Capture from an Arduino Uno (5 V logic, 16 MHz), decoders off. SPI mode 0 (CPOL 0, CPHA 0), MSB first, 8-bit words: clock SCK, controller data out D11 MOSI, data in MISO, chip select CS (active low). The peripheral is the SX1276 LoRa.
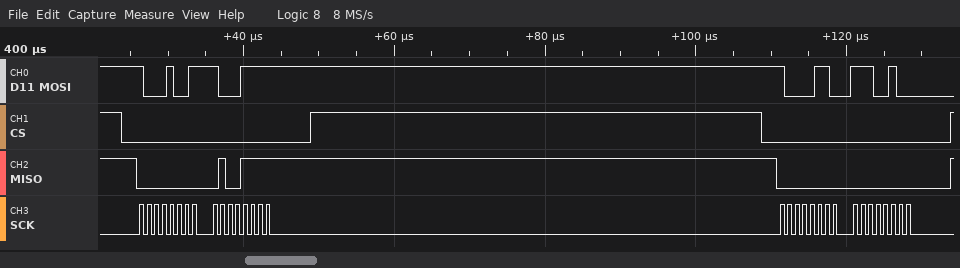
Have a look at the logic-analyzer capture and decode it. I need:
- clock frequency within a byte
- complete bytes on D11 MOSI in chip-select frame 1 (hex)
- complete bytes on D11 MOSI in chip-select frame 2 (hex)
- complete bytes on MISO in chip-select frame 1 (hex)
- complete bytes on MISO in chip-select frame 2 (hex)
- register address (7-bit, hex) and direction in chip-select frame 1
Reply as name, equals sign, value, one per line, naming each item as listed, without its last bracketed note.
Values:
clock frequency within a byte = 1 MHz
complete bytes on D11 MOSI in chip-select frame 1 = 89 8F
complete bytes on D11 MOSI in chip-select frame 2 = 86 E4
complete bytes on MISO in chip-select frame 1 = 00 4F
complete bytes on MISO in chip-select frame 2 = 00 00
register address (7-bit, hex) and direction in chip-select frame 1 = 0x09 write
